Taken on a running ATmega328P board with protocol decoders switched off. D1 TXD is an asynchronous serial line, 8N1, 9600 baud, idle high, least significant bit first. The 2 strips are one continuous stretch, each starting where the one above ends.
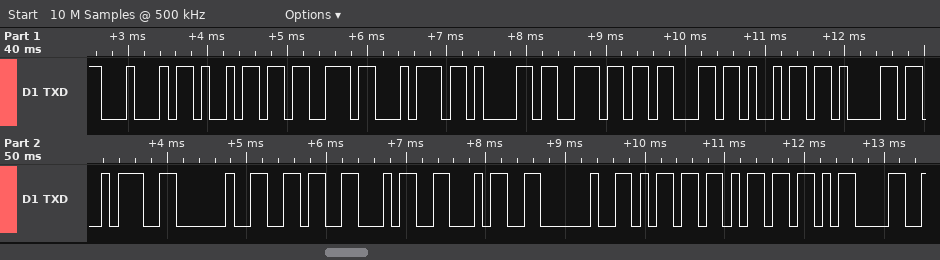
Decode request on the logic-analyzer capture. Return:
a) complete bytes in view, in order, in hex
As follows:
44 69 73 74 61 6E 63 69 61 3A 20 36 34 34 20 6D 6D 0D
